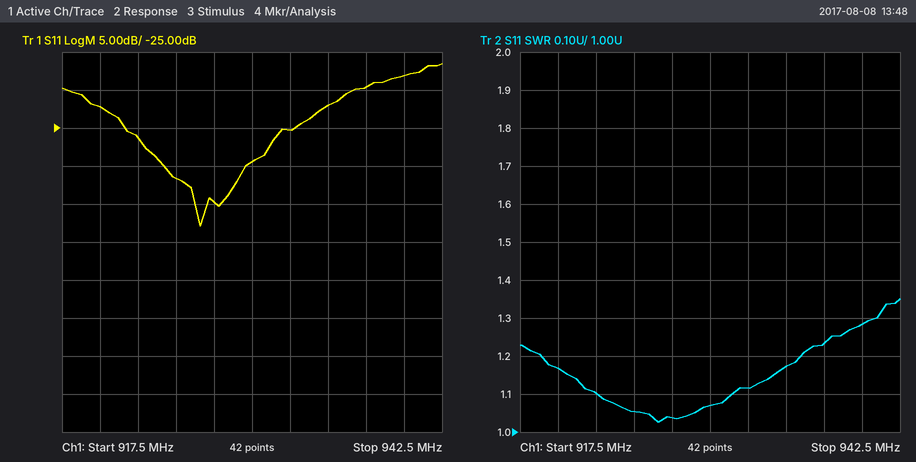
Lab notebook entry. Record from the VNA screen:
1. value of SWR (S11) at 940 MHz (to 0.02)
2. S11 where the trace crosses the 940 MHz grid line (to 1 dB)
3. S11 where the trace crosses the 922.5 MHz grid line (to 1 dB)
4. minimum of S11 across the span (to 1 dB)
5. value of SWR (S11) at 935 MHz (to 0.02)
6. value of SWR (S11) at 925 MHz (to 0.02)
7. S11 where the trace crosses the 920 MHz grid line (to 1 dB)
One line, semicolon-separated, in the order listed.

1.28; -18 dB; -26 dB; -38 dB; 1.18; 1.06; -22 dB
